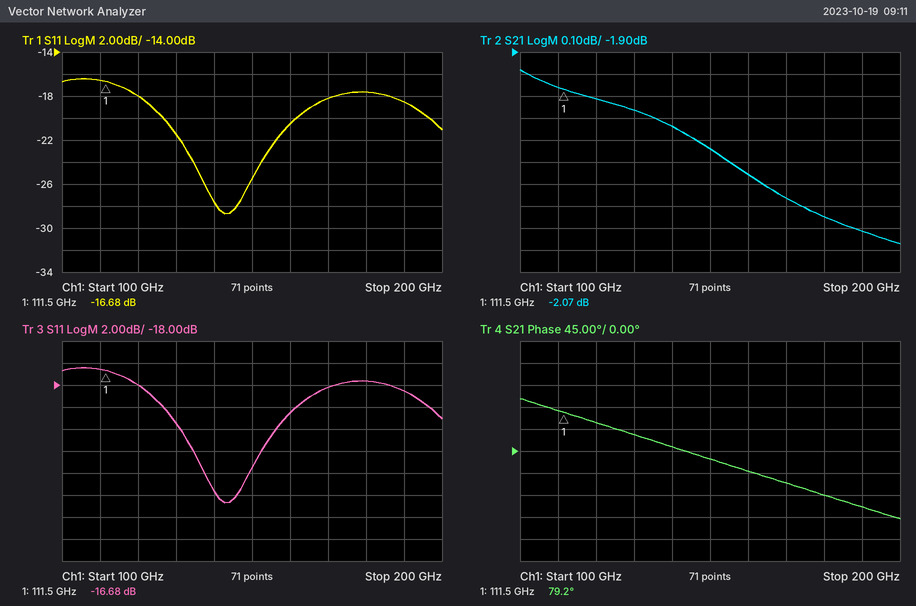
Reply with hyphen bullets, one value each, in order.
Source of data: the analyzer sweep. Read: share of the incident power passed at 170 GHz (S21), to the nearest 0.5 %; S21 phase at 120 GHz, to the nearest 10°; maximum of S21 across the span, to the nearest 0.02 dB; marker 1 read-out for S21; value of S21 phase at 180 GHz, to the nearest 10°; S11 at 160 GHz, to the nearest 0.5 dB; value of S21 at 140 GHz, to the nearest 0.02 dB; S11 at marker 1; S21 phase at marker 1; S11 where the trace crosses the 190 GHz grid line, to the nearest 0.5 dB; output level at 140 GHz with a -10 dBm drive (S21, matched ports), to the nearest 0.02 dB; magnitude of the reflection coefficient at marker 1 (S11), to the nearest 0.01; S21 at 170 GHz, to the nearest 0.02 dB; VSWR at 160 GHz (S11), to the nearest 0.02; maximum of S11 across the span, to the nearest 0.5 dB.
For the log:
- 55.5 %
- 60°
- -1.98 dB
- -2.07 dB
- -90°
- -20.5 dB
- -2.24 dB
- -16.68 dB
- 79.2°
- -18.5 dB
- -12.24 dBm
- 0.15
- -2.56 dB
- 1.20
- -16.5 dB
